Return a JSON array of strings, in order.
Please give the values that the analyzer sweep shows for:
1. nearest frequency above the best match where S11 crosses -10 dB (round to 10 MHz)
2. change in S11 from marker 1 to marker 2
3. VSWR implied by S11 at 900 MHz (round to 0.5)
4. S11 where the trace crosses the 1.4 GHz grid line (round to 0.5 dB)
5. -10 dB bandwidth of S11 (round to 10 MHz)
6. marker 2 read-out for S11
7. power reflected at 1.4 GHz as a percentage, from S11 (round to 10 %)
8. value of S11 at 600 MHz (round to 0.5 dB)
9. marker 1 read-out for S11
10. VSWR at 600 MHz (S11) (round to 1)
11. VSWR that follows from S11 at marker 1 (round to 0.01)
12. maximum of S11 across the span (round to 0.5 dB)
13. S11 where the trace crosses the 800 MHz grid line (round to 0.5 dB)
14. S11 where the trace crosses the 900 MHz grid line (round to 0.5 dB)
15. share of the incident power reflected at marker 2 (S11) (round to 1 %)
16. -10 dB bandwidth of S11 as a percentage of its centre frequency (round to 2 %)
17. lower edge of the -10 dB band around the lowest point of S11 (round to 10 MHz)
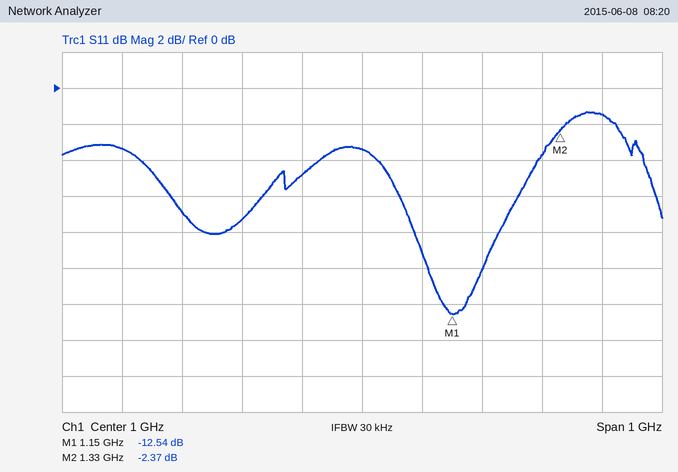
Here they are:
["1.20 GHz", "10.17 dB", "3.5", "-1.5 dB", "90 MHz", "-2.37 dB", "70 %", "-3.5 dB", "-12.54 dB", "5", "1.62", "-1.5 dB", "-7.5 dB", "-5.0 dB", "58 %", "8 %", "1.11 GHz"]
